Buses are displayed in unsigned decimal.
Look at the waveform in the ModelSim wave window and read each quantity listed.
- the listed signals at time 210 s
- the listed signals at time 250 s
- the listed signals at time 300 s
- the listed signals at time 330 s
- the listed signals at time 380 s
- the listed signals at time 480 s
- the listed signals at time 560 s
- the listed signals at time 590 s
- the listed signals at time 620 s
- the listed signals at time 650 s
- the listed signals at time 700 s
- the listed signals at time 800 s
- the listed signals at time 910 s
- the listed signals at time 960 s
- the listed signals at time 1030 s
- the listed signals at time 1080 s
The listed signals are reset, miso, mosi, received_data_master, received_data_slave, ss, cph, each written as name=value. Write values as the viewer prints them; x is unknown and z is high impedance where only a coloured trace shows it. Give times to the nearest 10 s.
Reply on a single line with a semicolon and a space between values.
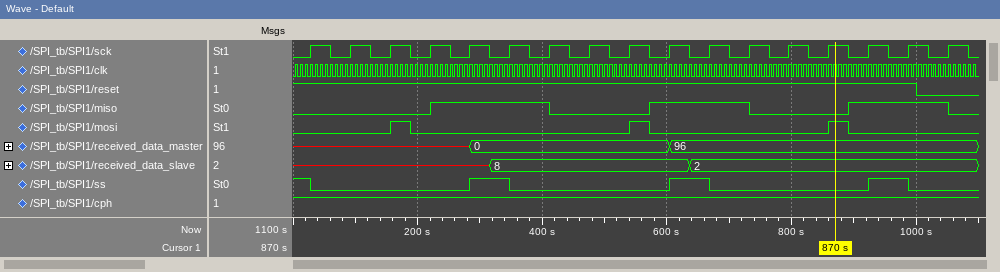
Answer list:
reset=1, miso=0, mosi=0, received_data_master=x, received_data_slave=x, ss=0, cph=1; reset=1, miso=1, mosi=0, received_data_master=x, received_data_slave=x, ss=0, cph=1; reset=1, miso=1, mosi=0, received_data_master=0, received_data_slave=x, ss=1, cph=1; reset=1, miso=1, mosi=0, received_data_master=0, received_data_slave=8, ss=1, cph=1; reset=1, miso=1, mosi=0, received_data_master=0, received_data_slave=8, ss=0, cph=1; reset=1, miso=0, mosi=0, received_data_master=0, received_data_slave=8, ss=0, cph=1; reset=1, miso=0, mosi=1, received_data_master=0, received_data_slave=8, ss=0, cph=1; reset=1, miso=1, mosi=0, received_data_master=0, received_data_slave=8, ss=0, cph=1; reset=1, miso=1, mosi=0, received_data_master=96, received_data_slave=8, ss=1, cph=1; reset=1, miso=1, mosi=0, received_data_master=96, received_data_slave=2, ss=1, cph=1; reset=1, miso=1, mosi=0, received_data_master=96, received_data_slave=2, ss=0, cph=1; reset=1, miso=0, mosi=0, received_data_master=96, received_data_slave=2, ss=0, cph=1; reset=1, miso=1, mosi=0, received_data_master=96, received_data_slave=2, ss=0, cph=1; reset=1, miso=1, mosi=0, received_data_master=96, received_data_slave=2, ss=1, cph=1; reset=0, miso=1, mosi=0, received_data_master=96, received_data_slave=2, ss=0, cph=1; reset=0, miso=0, mosi=0, received_data_master=96, received_data_slave=2, ss=0, cph=1
